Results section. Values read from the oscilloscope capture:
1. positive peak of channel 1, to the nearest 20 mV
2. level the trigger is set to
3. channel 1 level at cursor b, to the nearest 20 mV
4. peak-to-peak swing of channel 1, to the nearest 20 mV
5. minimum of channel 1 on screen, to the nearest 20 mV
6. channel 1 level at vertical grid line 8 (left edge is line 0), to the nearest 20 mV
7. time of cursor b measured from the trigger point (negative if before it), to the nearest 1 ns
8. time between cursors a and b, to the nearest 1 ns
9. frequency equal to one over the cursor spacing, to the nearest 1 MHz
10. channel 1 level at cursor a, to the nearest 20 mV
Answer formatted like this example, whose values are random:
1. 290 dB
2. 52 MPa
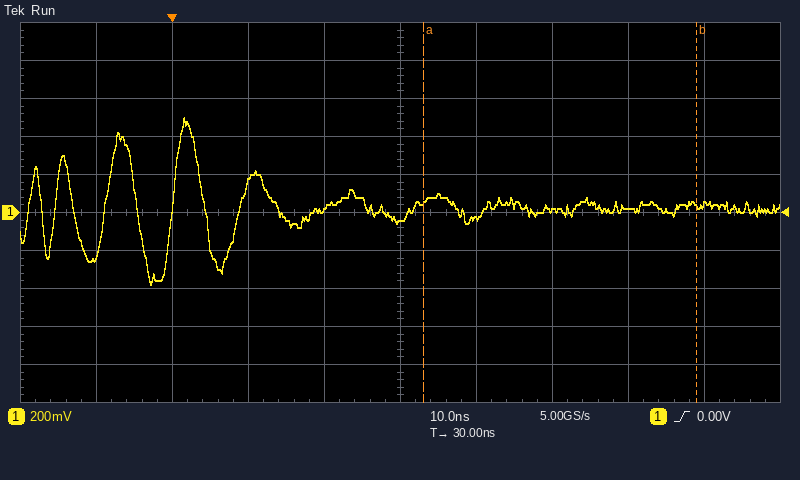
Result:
1. 500 mV
2. 0.00 V
3. 40 mV
4. 880 mV
5. -380 mV
6. 20 mV
7. +69 ns
8. 36 ns
9. 28 MHz
10. 60 mV
